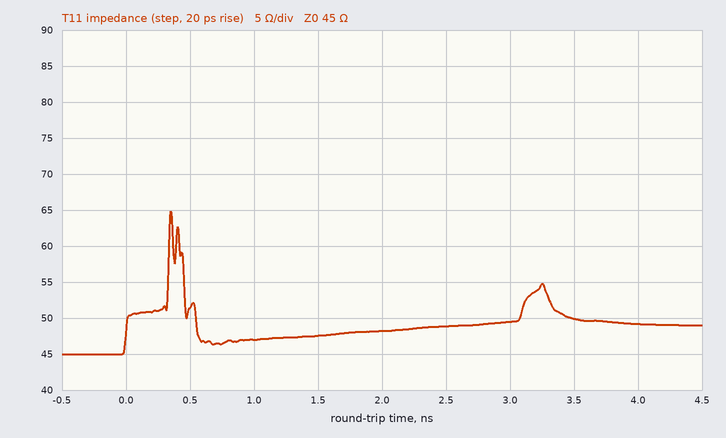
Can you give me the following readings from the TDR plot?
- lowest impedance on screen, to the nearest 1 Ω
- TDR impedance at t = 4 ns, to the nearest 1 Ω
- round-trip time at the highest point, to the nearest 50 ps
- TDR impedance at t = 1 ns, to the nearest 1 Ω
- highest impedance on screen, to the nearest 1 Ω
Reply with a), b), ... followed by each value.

a) 45 Ω
b) 49 Ω
c) 350 ps
d) 47 Ω
e) 65 Ω
